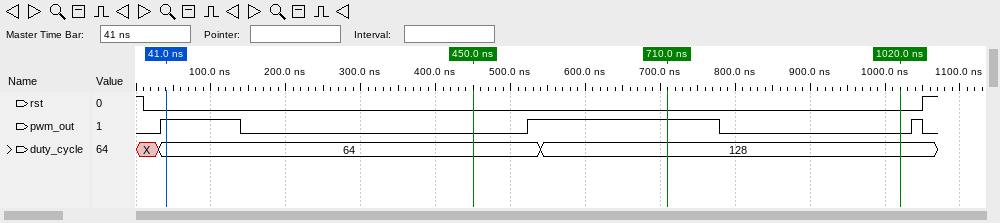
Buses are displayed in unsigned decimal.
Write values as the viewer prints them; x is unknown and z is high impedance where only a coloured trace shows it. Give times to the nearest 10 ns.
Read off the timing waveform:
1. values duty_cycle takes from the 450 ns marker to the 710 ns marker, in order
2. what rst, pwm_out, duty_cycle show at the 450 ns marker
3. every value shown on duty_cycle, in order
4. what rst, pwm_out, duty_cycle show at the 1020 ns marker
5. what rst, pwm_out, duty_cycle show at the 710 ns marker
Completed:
64, 128
rst=0, pwm_out=0, duty_cycle=64
X, 64, 128
rst=0, pwm_out=0, duty_cycle=128
rst=0, pwm_out=1, duty_cycle=128
